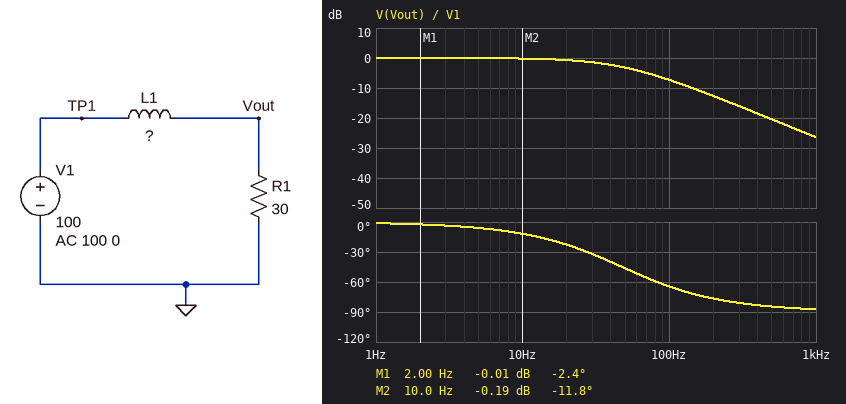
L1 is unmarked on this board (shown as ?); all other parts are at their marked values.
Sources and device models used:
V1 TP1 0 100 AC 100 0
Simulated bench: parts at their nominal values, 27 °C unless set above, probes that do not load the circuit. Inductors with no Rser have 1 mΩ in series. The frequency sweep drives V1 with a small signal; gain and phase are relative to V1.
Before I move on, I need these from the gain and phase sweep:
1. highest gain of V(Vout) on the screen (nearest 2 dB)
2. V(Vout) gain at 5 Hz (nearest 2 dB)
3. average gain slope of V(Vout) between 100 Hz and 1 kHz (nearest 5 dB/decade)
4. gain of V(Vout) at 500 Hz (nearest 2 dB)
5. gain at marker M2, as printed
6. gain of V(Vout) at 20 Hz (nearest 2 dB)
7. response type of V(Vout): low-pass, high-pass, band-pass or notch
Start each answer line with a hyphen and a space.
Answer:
- 0 dB
- 0 dB
- -20 dB/decade
- -20 dB
- -0.19 dB
- 0 dB
- low-pass
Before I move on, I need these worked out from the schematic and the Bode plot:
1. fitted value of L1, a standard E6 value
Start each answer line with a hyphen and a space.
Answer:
- 100 mH
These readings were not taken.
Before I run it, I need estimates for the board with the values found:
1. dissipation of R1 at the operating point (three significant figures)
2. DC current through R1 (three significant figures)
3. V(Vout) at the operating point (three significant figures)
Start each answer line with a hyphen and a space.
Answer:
- 333 W
- 3.33 A
- 100 V
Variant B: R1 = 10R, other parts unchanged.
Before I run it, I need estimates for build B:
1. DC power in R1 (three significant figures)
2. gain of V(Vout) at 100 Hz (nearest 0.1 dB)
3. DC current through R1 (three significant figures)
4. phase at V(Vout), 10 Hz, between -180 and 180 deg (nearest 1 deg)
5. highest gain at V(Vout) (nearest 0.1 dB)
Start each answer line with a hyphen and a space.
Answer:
- 1.00 kW
- -16.1 dB
- 10.0 A
- -32 deg
- 0 dB
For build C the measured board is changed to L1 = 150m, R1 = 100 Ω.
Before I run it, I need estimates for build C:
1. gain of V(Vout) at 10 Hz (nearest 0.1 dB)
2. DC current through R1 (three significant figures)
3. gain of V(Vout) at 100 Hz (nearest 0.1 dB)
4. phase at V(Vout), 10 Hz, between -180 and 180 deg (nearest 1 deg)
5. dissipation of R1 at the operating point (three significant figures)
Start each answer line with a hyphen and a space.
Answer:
- 0 dB
- 1.00 A
- -2.8 dB
- -5 deg
- 100 W
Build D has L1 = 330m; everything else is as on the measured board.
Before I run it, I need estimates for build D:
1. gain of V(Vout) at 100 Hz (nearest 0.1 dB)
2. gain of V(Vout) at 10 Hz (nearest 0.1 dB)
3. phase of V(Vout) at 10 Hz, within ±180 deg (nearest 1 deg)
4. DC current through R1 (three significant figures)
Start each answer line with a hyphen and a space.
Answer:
- -16.9 dB
- -1.7 dB
- -35 deg
- 3.33 A
